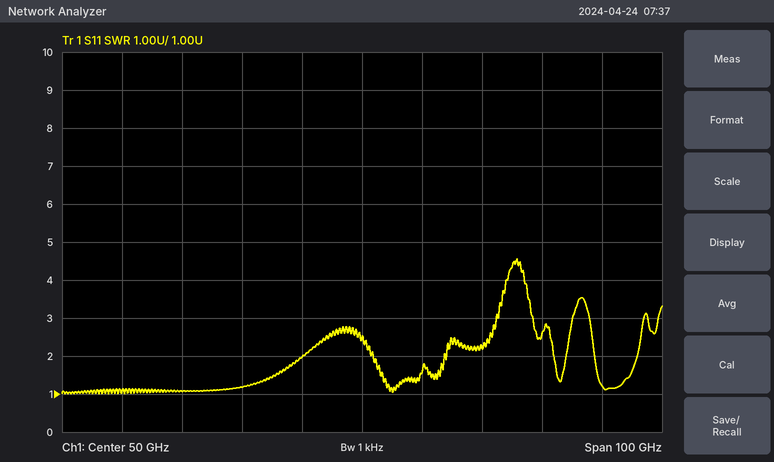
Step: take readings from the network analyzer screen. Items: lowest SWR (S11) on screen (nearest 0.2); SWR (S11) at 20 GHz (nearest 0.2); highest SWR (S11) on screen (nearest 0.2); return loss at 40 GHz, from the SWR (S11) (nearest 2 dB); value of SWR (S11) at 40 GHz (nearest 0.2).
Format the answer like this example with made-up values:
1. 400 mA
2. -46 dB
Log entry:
1. 1.0
2. 1.0
3. 4.6
4. 10 dB
5. 2.0
